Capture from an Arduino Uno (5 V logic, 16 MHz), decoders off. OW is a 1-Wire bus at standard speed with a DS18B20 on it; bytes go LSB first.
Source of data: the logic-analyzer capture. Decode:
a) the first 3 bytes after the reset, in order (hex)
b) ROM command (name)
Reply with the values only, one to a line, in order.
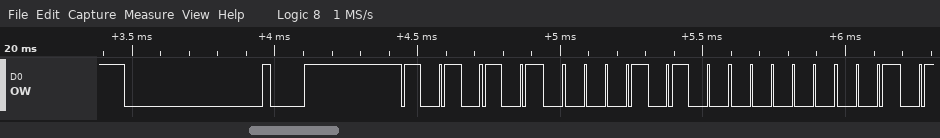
55 28 80
Match ROM
